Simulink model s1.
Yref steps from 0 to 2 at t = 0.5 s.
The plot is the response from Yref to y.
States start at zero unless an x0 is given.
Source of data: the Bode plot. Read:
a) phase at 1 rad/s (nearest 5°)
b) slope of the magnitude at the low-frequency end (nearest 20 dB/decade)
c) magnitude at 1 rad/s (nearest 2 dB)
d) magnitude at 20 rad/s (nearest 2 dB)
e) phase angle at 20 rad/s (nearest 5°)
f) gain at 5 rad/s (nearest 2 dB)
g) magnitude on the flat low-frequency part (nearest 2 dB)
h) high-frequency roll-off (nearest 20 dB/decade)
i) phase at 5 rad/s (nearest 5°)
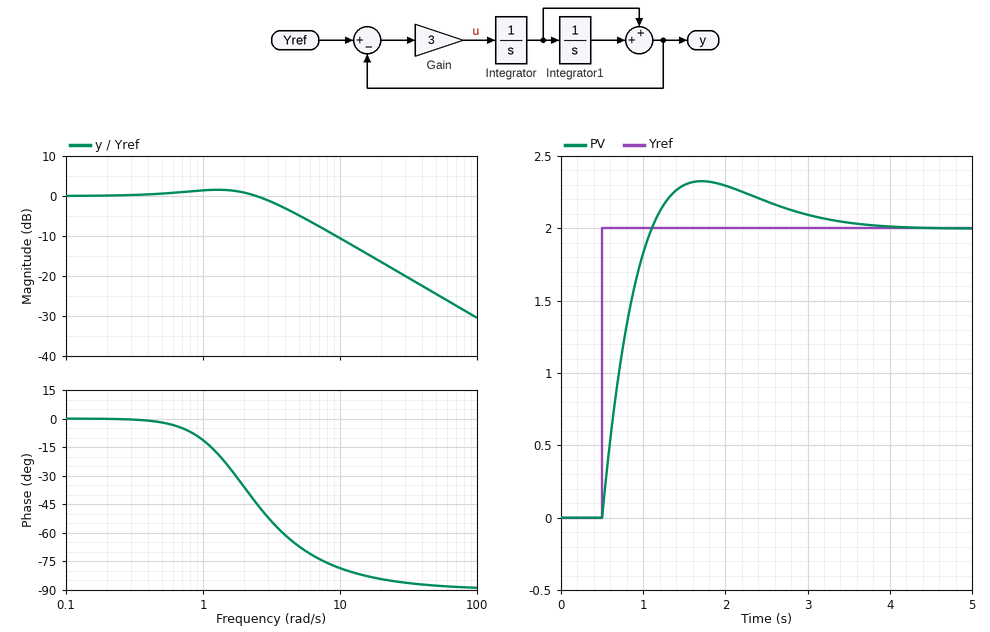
-10°
0 dB/decade
2 dB
-16 dB
-85°
-4 dB
0 dB
-20 dB/decade
-65°
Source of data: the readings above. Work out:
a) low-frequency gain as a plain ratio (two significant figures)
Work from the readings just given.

1.0
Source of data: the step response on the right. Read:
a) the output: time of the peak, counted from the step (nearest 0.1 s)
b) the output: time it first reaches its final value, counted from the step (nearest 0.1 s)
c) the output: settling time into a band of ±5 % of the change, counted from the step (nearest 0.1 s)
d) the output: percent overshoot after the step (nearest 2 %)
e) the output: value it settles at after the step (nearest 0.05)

1.2 s
0.6 s
2.5 s
16 %
2.00
